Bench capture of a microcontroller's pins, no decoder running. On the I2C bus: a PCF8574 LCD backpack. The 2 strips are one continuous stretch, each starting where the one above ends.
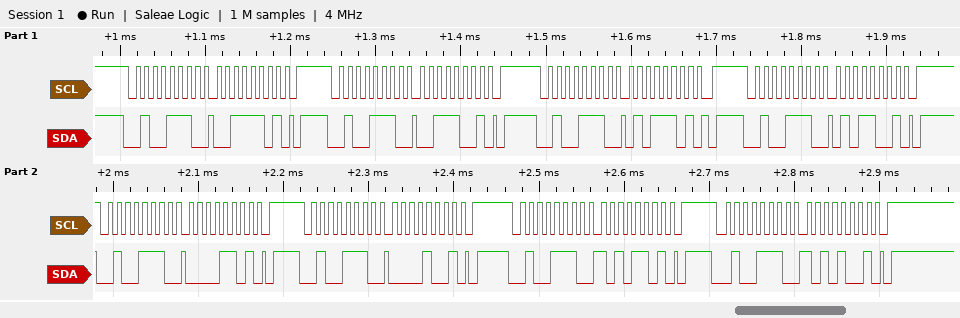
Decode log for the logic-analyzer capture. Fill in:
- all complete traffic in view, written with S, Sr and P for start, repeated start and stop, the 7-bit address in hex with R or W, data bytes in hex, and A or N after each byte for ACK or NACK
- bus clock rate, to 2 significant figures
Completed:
S 27W A 3D A P S 27W A 39 A P S 27W A 5D A P S 27W A 59 A P S 27W A 0D A P S 27W A 09 A P S 27W A AD A P S 27W A A9 A P
100 kHz
